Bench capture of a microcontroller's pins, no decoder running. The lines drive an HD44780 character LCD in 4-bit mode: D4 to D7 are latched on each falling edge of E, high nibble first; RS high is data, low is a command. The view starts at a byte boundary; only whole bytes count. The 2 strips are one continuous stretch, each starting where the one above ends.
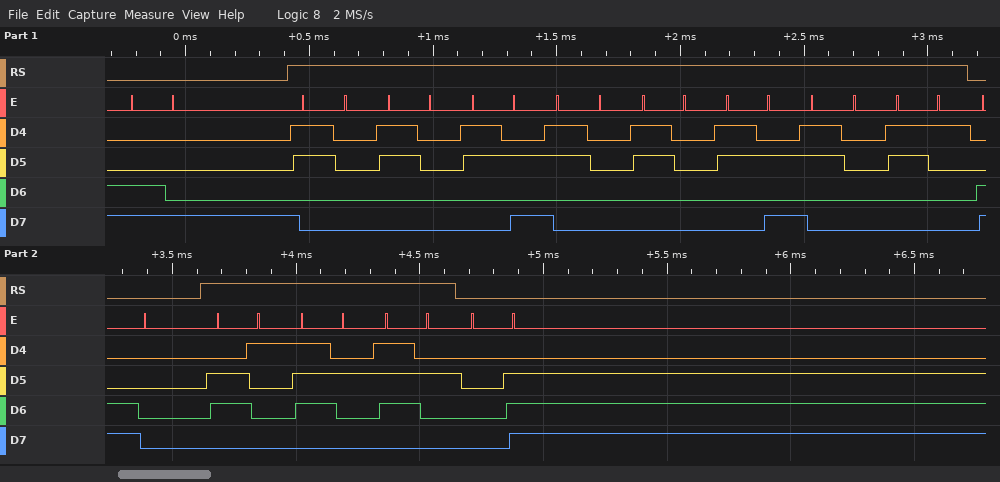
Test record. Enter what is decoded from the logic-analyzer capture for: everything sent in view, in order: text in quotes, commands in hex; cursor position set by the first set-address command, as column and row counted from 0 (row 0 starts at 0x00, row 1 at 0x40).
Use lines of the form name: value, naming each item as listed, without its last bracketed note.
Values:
everything sent in view, in order: text in quotes, commands in hex: 0xC8 "00:00:01" 0xC0 "arr" 0x0E
cursor position set by the first set-address command, as column and row counted from 0: column 8, row 1
